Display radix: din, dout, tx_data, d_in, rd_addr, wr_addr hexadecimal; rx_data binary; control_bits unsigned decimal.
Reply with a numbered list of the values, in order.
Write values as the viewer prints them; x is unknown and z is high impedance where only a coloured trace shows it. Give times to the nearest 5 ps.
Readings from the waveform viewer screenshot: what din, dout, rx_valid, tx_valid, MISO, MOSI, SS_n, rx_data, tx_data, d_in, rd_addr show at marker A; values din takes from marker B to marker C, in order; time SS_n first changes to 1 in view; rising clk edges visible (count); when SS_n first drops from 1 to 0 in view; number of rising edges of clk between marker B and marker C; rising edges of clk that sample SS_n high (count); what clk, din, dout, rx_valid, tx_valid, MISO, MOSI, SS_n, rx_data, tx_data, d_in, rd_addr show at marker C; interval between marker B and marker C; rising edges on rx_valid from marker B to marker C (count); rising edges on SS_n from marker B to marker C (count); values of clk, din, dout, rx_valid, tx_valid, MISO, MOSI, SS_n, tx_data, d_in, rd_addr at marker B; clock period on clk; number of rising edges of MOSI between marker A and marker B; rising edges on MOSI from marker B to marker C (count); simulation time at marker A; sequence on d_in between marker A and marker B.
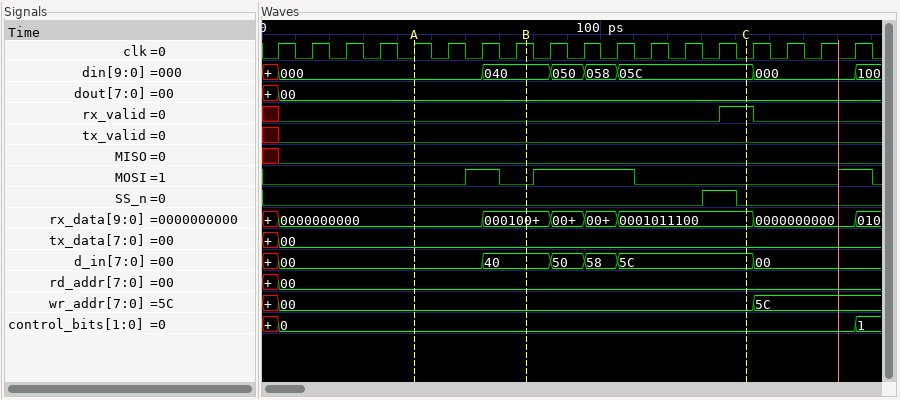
1. din=000, dout=00, rx_valid=0, tx_valid=0, MISO=0, MOSI=0, SS_n=0, rx_data=0000000000, tx_data=00, d_in=00, rd_addr=00
2. 040, 050, 058, 05C
3. 130 ps
4. 18
5. 140 ps
6. 6
7. 1
8. clk=0, din=05C, dout=00, rx_valid=1, tx_valid=0, MISO=0, MOSI=0, SS_n=0, rx_data=0001011100, tx_data=00, d_in=5C, rd_addr=00
9. 65 ps
10. 1
11. 1
12. clk=1, din=040, dout=00, rx_valid=0, tx_valid=0, MISO=0, MOSI=0, SS_n=0, tx_data=00, d_in=40, rd_addr=00
13. 10 ps
14. 1
15. 1
16. 45 ps
17. 00, 40
